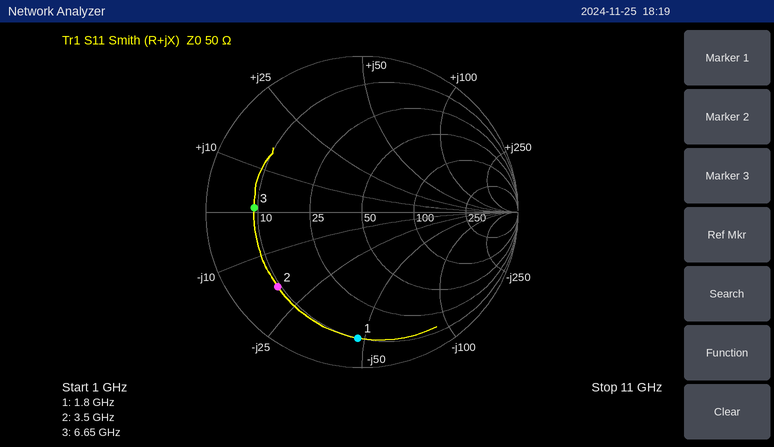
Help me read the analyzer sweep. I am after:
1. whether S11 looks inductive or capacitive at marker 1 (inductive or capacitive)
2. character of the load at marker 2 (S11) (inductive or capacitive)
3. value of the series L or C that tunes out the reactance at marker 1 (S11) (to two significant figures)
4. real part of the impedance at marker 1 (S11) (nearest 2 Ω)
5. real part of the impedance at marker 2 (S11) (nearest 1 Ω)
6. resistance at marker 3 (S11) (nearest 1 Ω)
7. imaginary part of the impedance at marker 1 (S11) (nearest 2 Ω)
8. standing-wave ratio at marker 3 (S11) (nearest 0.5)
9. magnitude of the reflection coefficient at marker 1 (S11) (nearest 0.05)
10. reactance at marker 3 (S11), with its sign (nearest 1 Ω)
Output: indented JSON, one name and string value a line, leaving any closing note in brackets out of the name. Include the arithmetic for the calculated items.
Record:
{
  "whether S11 looks inductive or capacitive at marker 1": "capacitive",
  "character of the load at marker 2 (S11)": "capacitive",
  "value of the series L or C that tunes out the reactance at marker 1 (S11)": "L = 48 Ω/(2π × 1.8 GHz) ≈ 4.2 nH",
  "real part of the impedance at marker 1 (S11)": "10 Ω",
  "real part of the impedance at marker 2 (S11)": "9 Ω",
  "resistance at marker 3 (S11)": "9 Ω",
  "imaginary part of the impedance at marker 1 (S11)": "-48 Ω",
  "standing-wave ratio at marker 3 (S11)": "5.5",
  "magnitude of the reflection coefficient at marker 1 (S11)": "0.80",
  "reactance at marker 3 (S11), with its sign": "+1 Ω"
}
